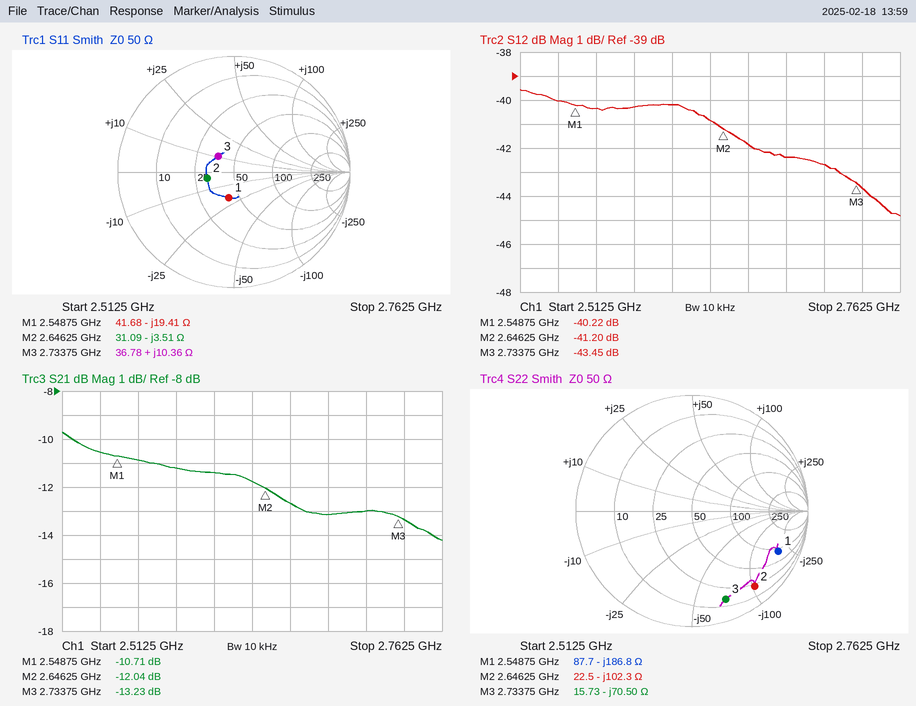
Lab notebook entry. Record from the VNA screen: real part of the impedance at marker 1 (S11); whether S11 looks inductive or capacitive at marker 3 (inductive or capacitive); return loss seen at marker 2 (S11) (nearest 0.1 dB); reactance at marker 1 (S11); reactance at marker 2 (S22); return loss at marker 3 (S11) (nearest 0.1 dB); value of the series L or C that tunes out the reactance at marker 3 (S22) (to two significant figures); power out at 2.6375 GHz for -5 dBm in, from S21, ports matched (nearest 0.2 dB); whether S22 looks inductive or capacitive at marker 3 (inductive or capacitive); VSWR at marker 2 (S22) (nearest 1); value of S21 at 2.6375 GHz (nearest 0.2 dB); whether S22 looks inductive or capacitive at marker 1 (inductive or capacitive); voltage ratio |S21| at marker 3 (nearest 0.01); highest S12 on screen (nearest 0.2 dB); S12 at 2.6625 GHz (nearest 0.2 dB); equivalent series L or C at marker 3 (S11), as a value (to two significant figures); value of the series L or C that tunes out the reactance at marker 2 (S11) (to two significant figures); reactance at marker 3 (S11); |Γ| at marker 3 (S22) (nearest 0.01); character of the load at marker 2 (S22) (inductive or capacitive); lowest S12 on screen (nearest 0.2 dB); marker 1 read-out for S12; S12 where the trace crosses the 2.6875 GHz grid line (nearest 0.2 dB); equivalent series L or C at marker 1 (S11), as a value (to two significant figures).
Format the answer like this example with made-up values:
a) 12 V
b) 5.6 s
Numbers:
a) 41.68 Ω
b) inductive
c) 12.5 dB
d) -19.41 Ω
e) -102.3 Ω
f) 14.3 dB
g) 4.1 nH
h) -16.8 dBm
i) capacitive
j) 12
k) -11.8 dB
l) capacitive
m) 0.22
n) -39.6 dB
o) -41.8 dB
p) 600 pH
q) 210 pH
r) +10.36 Ω
s) 0.81
t) capacitive
u) -44.8 dB
v) -40.22 dB
w) -42.4 dB
x) 3.2 pF
